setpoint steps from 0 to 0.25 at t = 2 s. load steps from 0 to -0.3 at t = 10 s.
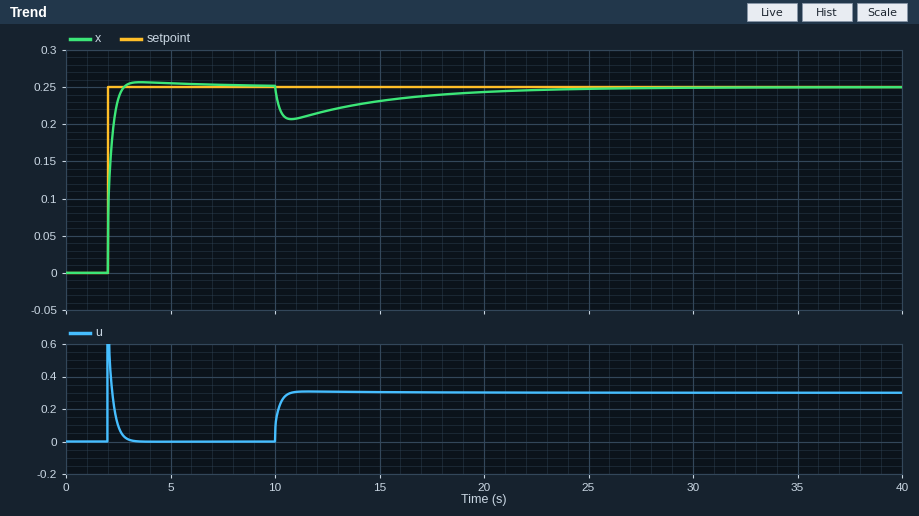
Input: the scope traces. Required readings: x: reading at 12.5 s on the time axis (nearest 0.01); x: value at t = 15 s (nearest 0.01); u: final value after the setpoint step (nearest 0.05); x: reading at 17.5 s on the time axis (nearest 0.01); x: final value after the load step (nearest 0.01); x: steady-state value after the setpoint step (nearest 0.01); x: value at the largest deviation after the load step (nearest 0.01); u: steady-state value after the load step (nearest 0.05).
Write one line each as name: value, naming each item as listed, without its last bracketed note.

x: reading at 12.5 s on the time axis: 0.22
x: value at t = 15 s: 0.23
u: final value after the setpoint step: 0.00
x: reading at 17.5 s on the time axis: 0.24
x: final value after the load step: 0.25
x: steady-state value after the setpoint step: 0.25
x: value at the largest deviation after the load step: 0.21
u: steady-state value after the load step: 0.30
